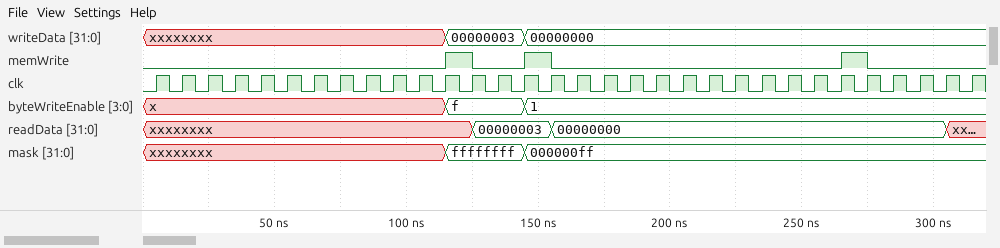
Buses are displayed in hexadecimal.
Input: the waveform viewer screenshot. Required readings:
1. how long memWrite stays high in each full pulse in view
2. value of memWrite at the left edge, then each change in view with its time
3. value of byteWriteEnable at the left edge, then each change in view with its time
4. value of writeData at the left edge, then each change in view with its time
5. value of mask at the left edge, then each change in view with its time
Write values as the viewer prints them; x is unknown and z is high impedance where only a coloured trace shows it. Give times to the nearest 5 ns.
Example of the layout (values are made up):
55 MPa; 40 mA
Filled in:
10 ns, 10 ns, 10 ns; 0, 1 at 115 ns, 0 at 125 ns, 1 at 145 ns, 0 at 155 ns, 1 at 265 ns, 0 at 275 ns; x, f at 115 ns, 1 at 145 ns; xxxxxxxx, 00000003 at 115 ns, 00000000 at 145 ns; xxxxxxxx, ffffffff at 115 ns, 000000ff at 145 ns
